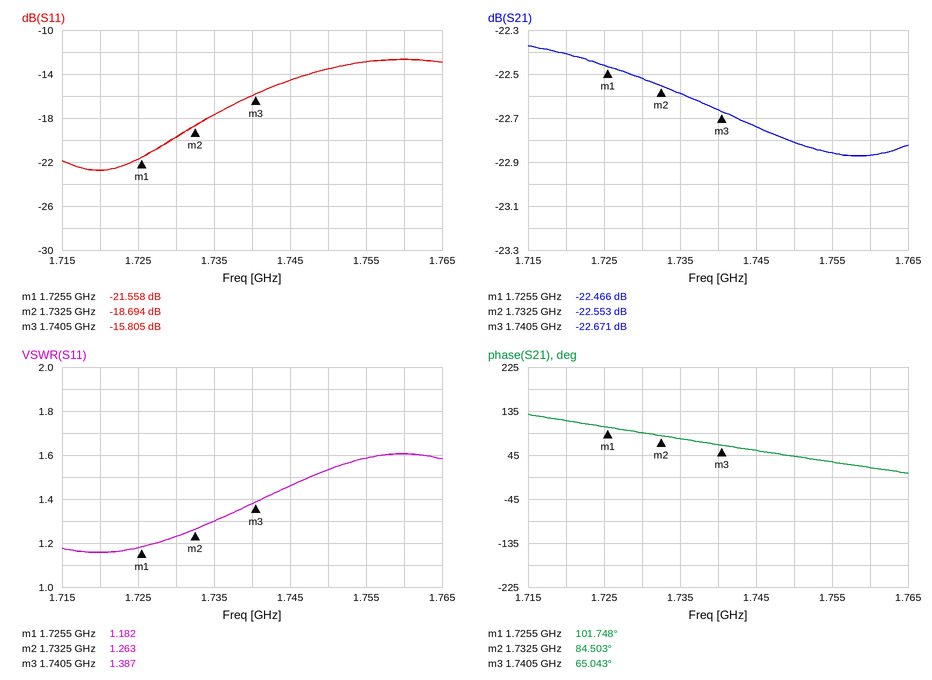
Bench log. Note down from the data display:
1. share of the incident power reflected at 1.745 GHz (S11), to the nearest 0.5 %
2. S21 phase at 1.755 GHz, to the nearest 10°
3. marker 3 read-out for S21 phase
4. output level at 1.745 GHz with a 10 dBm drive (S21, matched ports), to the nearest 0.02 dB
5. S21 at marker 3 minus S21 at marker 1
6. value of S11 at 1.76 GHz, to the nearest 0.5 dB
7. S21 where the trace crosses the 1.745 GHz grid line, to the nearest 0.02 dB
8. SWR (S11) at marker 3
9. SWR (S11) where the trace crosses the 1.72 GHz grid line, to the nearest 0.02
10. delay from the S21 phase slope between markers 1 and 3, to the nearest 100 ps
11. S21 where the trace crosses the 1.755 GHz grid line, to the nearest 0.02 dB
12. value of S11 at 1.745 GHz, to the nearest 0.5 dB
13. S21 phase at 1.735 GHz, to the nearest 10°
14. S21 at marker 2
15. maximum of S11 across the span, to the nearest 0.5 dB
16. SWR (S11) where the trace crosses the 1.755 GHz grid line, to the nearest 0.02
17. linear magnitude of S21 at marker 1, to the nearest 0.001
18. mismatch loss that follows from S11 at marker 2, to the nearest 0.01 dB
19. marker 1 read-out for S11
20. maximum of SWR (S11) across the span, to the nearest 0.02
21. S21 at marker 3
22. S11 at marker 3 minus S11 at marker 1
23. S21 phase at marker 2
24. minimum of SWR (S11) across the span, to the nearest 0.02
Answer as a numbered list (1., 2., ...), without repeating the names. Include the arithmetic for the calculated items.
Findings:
1. 10^(-14.5/10) ≈ 3.5 %
2. 30°
3. 65.043°
4. 10 dBm + (-22.74 dB) = -12.74 dBm
5. -22.671 − (-22.466) = -0.205 dB
6. -12.5 dB
7. -22.74 dB
8. 1.387
9. 1.16
10. −(65.043° − (101.748°))/(360° × 15 MHz) ≈ 6.8 ns
11. -22.86 dB
12. -14.5 dB
13. 80°
14. -22.553 dB
15. -12.5 dB
16. 1.58
17. 10^(-22.466/20) ≈ 0.075
18. −10 log10(1 − 10^(-18.694/10)) ≈ 0.06 dB
19. -21.558 dB
20. 1.60
21. -22.671 dB
22. -15.805 − (-21.558) = 5.753 dB
23. 84.503°
24. 1.16
